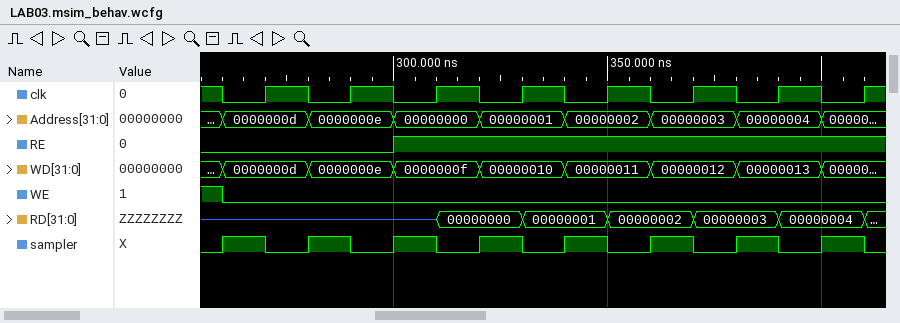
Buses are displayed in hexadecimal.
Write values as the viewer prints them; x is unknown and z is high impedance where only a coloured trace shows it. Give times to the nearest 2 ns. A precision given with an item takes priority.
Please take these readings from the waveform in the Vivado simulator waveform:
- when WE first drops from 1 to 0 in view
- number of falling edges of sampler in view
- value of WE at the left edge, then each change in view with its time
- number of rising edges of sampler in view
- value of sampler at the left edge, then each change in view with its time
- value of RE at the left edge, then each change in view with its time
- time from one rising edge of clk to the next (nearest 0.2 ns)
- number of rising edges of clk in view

260 ns
8
1, 0 at 260 ns
8
0, 1 at 260 ns, 0 at 270 ns, 1 at 280 ns, 0 at 290 ns, 1 at 300 ns, 0 at 310 ns, 1 at 320 ns, 0 at 330 ns, 1 at 340 ns, 0 at 350 ns, 1 at 360 ns, 0 at 370 ns, 1 at 380 ns, 0 at 390 ns, 1 at 400 ns, 0 at 410 ns
0, 1 at 300 ns
20 ns
8
